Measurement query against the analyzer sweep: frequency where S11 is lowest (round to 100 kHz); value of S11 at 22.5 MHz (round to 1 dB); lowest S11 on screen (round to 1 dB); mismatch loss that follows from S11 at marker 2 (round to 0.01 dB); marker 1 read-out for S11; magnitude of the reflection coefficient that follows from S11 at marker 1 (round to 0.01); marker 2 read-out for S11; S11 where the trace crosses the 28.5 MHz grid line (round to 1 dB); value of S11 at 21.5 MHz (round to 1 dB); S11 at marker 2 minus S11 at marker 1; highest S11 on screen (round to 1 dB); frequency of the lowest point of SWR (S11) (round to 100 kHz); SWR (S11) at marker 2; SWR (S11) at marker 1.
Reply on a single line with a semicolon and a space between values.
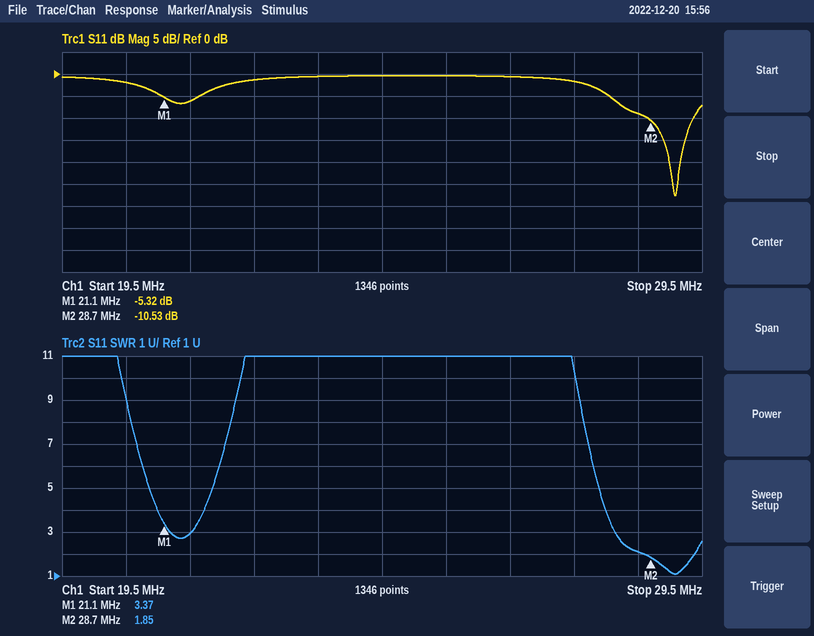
29.1 MHz; -1 dB; -28 dB; 0.40 dB; -5.32 dB; 0.54; -10.53 dB; -9 dB; -6 dB; -5.21 dB; 0 dB; 29.1 MHz; 1.85; 3.37
